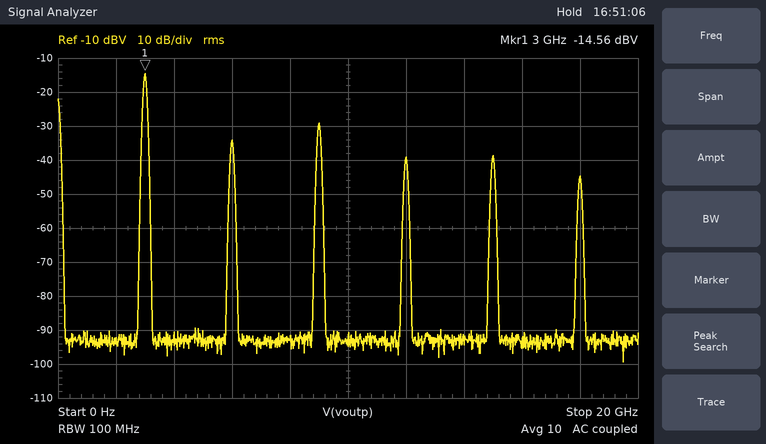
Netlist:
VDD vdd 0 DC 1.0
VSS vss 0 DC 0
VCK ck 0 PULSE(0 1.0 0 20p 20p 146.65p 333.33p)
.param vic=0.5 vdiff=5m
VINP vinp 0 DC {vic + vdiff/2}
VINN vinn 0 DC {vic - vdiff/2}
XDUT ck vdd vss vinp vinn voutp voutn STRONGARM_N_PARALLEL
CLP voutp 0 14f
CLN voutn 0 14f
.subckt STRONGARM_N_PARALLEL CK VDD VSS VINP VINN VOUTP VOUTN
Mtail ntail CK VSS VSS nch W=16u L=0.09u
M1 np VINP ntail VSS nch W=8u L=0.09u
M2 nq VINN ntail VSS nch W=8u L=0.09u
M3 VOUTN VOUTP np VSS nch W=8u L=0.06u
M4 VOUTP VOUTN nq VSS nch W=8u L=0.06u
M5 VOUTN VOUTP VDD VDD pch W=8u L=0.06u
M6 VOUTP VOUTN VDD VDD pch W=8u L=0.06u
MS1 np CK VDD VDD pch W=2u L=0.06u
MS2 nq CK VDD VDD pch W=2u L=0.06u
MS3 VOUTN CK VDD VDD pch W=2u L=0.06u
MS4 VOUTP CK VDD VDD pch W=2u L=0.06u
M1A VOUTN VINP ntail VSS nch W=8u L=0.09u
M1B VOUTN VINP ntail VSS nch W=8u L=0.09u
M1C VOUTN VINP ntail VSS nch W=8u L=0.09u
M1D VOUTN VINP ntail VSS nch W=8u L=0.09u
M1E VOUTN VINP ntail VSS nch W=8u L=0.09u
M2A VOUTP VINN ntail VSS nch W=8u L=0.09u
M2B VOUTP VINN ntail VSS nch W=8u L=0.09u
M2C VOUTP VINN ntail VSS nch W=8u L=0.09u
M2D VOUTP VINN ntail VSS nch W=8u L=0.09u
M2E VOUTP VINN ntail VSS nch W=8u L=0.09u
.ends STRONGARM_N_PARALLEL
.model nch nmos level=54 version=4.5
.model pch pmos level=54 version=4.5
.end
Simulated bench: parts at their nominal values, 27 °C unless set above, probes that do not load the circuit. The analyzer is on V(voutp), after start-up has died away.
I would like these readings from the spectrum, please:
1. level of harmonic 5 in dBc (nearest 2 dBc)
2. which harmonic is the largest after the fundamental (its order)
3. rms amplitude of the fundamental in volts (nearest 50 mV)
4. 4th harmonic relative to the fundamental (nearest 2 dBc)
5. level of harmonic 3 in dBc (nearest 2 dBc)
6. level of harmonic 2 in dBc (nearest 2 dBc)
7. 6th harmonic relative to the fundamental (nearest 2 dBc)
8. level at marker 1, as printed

-24 dBc
3
200 mV
-24 dBc
-14 dBc
-20 dBc
-30 dBc
-14.56 dBV
